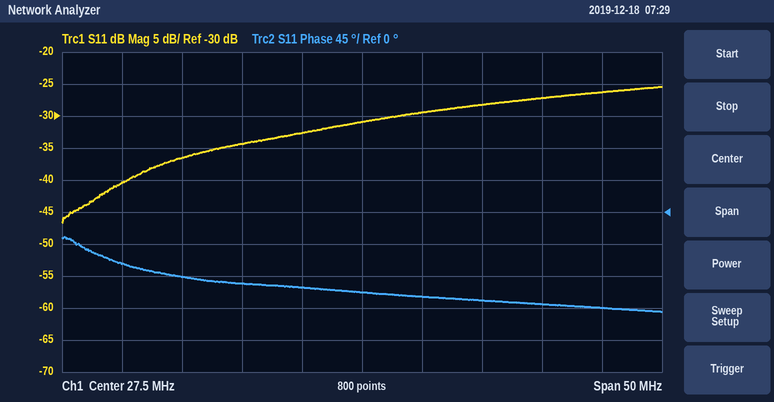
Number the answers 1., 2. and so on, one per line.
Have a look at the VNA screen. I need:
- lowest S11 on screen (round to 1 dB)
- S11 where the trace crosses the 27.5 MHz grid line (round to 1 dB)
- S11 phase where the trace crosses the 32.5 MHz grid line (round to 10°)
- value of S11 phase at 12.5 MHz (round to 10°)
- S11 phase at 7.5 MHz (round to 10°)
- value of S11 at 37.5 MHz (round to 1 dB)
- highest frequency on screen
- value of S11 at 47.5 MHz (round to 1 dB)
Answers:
1. -47 dB
2. -31 dB
3. -120°
4. -90°
5. -70°
6. -28 dB
7. 52.5 MHz
8. -26 dB
